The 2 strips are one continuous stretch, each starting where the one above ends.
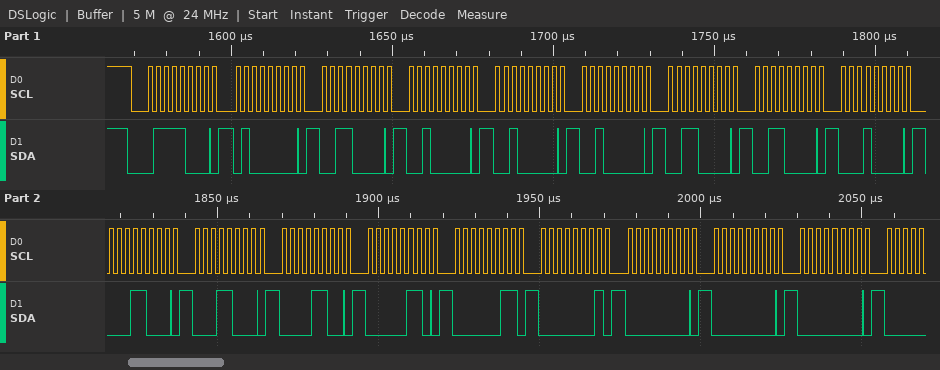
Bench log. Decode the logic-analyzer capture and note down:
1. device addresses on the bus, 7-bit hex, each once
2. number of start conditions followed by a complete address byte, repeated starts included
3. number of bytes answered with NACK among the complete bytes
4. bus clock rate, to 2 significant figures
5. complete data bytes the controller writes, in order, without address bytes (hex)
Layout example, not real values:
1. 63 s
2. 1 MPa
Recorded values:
1. 0x3C
2. 1
3. 0
4. 400 kHz
5. 40 30 20 20 20 30 30 10 18 18 0C 06 03 01 00 00 00
